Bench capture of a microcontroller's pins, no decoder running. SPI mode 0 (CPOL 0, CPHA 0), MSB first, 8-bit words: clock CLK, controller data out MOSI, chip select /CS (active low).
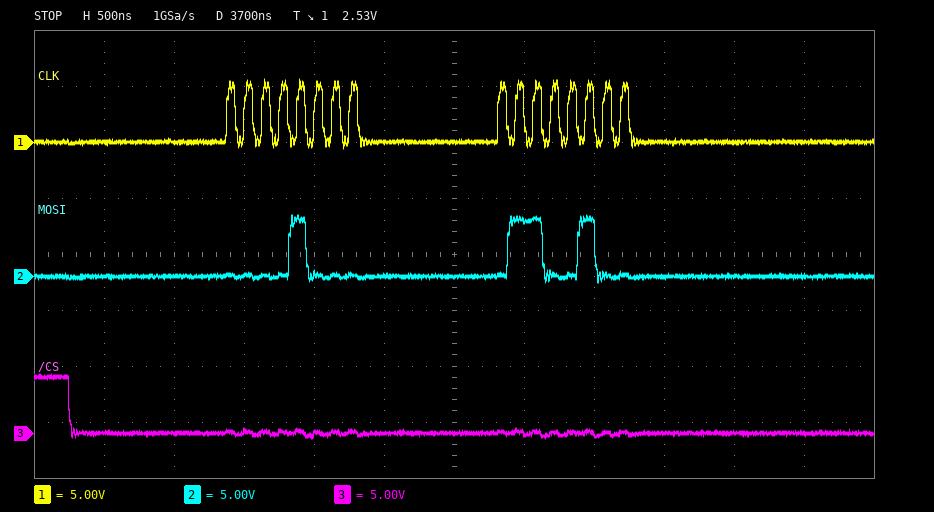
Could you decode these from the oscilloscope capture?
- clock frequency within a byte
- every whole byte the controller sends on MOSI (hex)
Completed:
8 MHz
08 64
